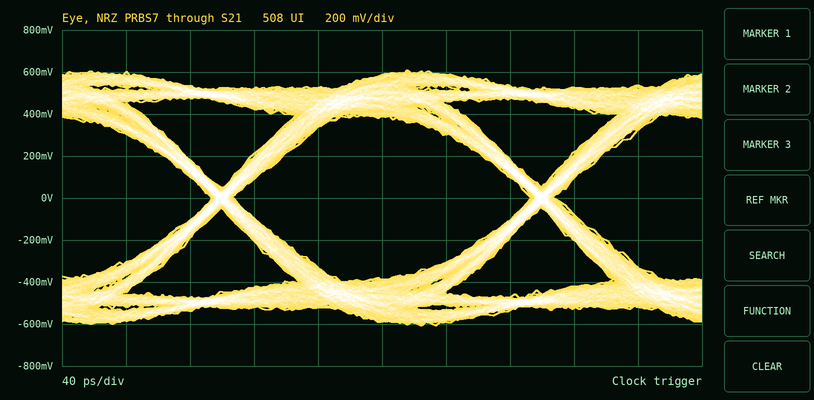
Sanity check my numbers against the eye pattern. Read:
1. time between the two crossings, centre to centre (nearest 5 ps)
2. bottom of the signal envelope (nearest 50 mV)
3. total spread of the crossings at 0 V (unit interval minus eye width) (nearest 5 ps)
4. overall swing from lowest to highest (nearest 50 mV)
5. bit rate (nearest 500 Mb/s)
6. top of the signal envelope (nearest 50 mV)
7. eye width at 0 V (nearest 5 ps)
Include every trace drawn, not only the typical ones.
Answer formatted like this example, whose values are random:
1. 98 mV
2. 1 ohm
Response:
1. 200 ps
2. -600 mV
3. 15 ps
4. 1.20 V
5. 5.0 Gb/s
6. 600 mV
7. 185 ps
